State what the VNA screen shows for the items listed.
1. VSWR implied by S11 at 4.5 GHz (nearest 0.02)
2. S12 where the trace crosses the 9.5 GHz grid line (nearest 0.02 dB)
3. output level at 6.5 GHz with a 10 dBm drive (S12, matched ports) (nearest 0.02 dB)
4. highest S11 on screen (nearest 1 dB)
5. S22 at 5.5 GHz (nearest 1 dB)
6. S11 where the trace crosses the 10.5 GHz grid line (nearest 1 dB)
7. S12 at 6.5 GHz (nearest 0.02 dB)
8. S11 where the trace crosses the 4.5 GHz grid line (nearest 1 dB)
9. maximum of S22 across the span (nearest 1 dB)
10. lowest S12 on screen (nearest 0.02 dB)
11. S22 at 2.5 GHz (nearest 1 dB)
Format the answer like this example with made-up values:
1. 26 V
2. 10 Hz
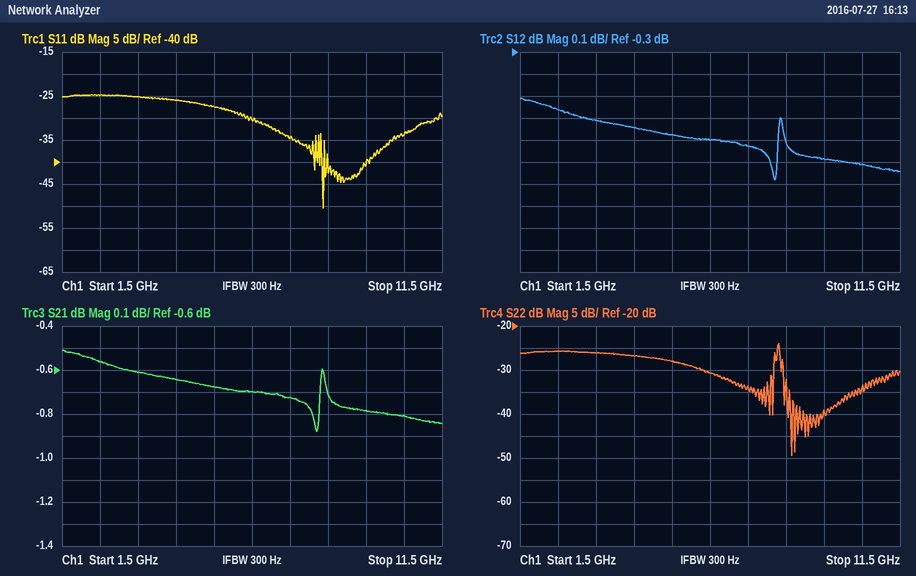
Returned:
1. 1.10
2. -0.78 dB
3. 9.30 dBm
4. -25 dB
5. -28 dB
6. -34 dB
7. -0.70 dB
8. -26 dB
9. -24 dB
10. -0.88 dB
11. -26 dB
